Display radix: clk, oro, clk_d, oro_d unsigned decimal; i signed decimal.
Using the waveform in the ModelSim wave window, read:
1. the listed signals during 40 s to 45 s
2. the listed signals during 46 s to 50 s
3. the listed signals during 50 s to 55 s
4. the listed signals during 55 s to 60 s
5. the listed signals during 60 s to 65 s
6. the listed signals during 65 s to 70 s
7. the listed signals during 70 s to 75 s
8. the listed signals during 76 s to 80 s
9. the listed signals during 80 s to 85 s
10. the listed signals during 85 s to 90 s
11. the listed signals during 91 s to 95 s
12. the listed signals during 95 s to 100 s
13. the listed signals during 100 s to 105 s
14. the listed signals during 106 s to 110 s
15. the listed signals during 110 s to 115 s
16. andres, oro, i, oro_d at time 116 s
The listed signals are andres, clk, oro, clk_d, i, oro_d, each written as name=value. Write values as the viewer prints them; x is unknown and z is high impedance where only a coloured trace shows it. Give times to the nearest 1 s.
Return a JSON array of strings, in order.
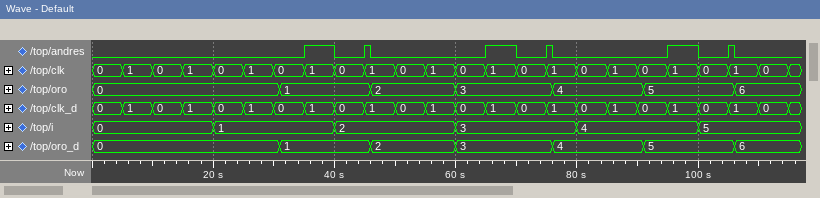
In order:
["andres=0, clk=0, oro=1, clk_d=0, i=2, oro_d=1", "andres=0, clk=1, oro=2, clk_d=1, i=2, oro_d=2", "andres=0, clk=0, oro=2, clk_d=0, i=2, oro_d=2", "andres=0, clk=1, oro=2, clk_d=1, i=2, oro_d=2", "andres=0, clk=0, oro=3, clk_d=0, i=3, oro_d=3", "andres=1, clk=1, oro=3, clk_d=1, i=3, oro_d=3", "andres=0, clk=0, oro=3, clk_d=0, i=3, oro_d=3", "andres=0, clk=1, oro=4, clk_d=1, i=3, oro_d=4", "andres=0, clk=0, oro=4, clk_d=0, i=4, oro_d=4", "andres=0, clk=1, oro=4, clk_d=1, i=4, oro_d=4", "andres=0, clk=0, oro=5, clk_d=0, i=4, oro_d=5", "andres=1, clk=1, oro=5, clk_d=1, i=4, oro_d=5", "andres=0, clk=0, oro=5, clk_d=0, i=5, oro_d=5", "andres=0, clk=1, oro=6, clk_d=1, i=5, oro_d=6", "andres=0, clk=0, oro=6, clk_d=0, i=5, oro_d=6", "andres=0, oro=6, i=5, oro_d=6"]
